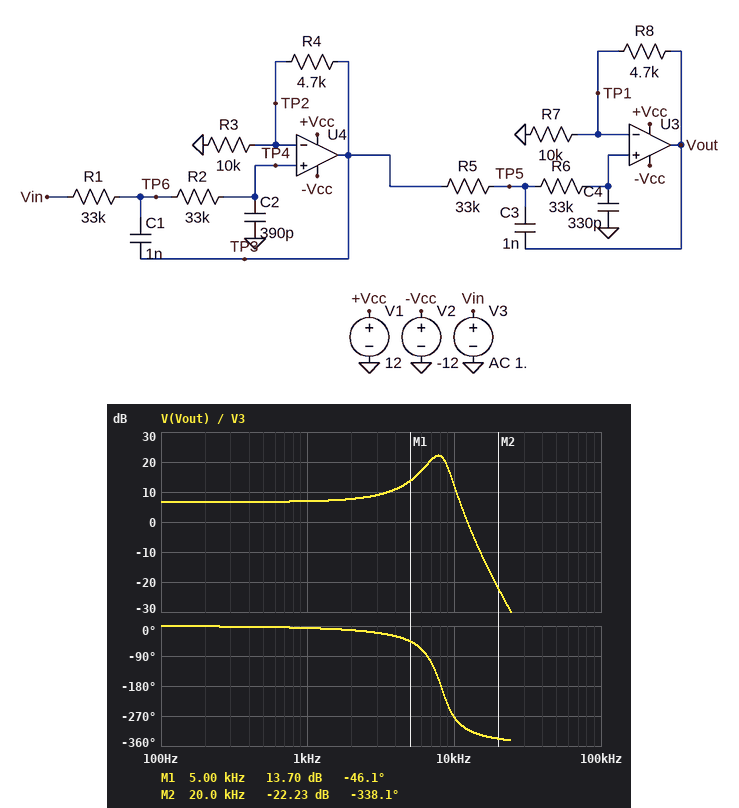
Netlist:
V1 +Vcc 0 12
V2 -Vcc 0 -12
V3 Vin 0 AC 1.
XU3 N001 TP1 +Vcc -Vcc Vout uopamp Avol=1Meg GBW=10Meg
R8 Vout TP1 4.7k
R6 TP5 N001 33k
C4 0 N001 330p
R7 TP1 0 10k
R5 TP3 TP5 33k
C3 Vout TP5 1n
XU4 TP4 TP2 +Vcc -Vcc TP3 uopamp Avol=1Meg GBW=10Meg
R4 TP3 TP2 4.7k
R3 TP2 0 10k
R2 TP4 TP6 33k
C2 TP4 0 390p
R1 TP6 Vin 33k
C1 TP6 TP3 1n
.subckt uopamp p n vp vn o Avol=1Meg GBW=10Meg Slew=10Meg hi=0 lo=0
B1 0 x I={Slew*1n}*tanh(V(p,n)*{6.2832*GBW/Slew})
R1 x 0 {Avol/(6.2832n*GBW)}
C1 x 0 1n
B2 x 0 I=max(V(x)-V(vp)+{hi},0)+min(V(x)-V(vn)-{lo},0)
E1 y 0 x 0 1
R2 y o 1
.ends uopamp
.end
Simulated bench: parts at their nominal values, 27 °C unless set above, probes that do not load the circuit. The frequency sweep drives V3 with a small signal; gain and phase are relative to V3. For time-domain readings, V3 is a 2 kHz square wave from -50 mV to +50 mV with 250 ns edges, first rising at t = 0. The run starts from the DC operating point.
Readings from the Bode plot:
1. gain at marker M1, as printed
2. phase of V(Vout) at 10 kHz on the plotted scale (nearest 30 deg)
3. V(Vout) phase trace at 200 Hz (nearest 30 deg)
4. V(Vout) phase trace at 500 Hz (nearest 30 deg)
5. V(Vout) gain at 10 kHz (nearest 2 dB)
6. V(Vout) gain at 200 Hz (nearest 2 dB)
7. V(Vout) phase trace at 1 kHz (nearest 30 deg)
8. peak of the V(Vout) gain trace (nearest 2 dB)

13.70 dB
-270 deg
0 deg
0 deg
12 dB
6 dB
0 deg
22 dB
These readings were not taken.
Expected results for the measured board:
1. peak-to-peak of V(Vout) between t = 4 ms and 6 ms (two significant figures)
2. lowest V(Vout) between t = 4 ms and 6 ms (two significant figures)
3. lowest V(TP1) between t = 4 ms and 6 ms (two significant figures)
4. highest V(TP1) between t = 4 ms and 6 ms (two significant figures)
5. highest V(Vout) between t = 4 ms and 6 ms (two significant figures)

580 mV
-290 mV
-200 mV
200 mV
290 mV
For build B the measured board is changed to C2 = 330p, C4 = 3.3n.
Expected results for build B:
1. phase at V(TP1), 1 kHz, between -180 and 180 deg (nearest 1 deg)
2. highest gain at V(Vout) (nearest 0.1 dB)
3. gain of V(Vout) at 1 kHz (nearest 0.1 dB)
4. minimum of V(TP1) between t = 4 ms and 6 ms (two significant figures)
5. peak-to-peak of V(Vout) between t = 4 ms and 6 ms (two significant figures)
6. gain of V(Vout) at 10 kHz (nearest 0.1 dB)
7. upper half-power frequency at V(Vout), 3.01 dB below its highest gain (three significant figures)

-58 deg
6.7 dB
3.1 dB
-42 mV
120 mV
-13.8 dB
880 Hz
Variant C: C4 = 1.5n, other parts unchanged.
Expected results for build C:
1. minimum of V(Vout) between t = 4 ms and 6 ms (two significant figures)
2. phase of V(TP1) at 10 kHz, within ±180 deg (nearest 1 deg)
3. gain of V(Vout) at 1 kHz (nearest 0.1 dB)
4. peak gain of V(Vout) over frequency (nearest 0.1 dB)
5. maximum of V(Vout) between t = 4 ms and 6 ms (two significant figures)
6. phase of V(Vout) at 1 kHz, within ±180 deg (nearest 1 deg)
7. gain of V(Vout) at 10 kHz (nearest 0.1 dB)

-110 mV
87 deg
6.2 dB
6.7 dB
110 mV
-33 deg
-10.3 dB
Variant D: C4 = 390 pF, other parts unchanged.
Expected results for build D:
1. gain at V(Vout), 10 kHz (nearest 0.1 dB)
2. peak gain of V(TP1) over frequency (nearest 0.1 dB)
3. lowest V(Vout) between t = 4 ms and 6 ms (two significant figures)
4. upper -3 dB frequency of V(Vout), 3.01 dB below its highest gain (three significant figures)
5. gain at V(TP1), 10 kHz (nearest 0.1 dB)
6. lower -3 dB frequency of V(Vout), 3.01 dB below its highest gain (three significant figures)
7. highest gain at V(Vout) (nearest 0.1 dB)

7.8 dB
16.1 dB
-290 mV
8.40 kHz
4.5 dB
5.81 kHz
19.4 dB
